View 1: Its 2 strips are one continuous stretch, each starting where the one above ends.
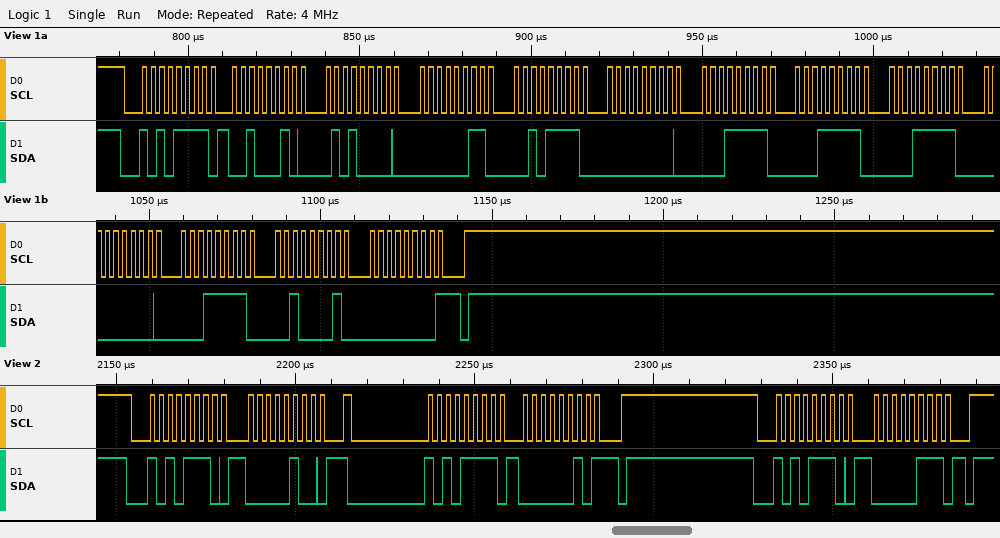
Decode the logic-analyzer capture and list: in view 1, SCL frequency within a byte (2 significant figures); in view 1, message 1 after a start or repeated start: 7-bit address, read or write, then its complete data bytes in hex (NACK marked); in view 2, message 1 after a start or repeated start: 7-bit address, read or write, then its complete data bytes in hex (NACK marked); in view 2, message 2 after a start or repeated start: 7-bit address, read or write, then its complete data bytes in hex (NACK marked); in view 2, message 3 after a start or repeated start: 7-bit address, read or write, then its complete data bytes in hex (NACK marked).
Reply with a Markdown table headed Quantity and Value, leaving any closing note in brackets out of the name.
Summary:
| Quantity | Value |
|---|---|
| in view 1, SCL frequency within a byte | 400 kHz |
| in view 1, message 1 after a start or repeated start: 7-bit address, read or write, then its complete data bytes in hex | 0x57 read: 22 50 03 2F 00 1F 1F 1F 00 1F 21 00 NACK |
| in view 2, message 1 after a start or repeated start: 7-bit address, read or write, then its complete data bytes in hex | 0x57 write: 04 |
| in view 2, message 2 after a start or repeated start: 7-bit address, read or write, then its complete data bytes in hex | 0x57 read: 02 NACK |
| in view 2, message 3 after a start or repeated start: 7-bit address, read or write, then its complete data bytes in hex | 0x57 write: 07 |
